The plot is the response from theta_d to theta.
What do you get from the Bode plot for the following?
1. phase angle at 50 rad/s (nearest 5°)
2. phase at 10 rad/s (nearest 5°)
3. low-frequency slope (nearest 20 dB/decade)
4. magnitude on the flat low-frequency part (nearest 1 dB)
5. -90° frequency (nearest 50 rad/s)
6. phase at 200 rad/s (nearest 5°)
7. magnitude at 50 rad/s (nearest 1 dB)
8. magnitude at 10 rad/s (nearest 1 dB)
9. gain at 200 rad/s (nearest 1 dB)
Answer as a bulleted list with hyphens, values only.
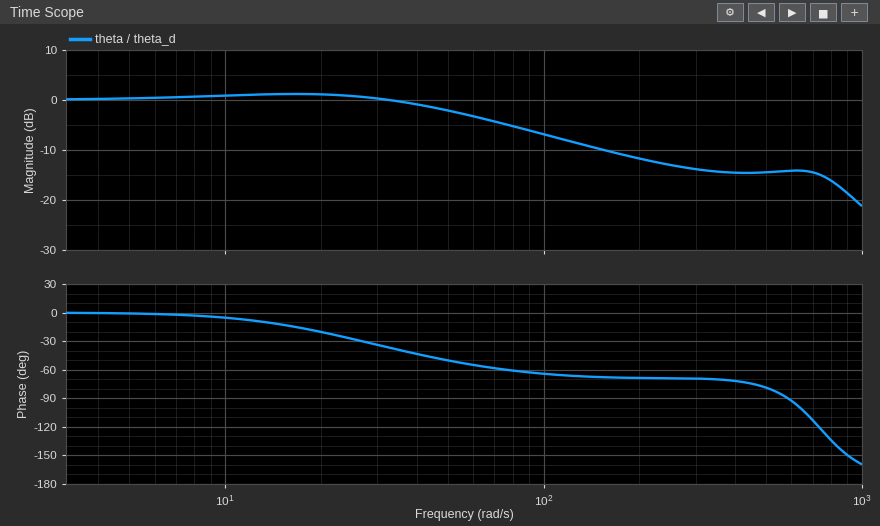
- -50°
- -5°
- 0 dB/decade
- 0 dB
- 600 rad/s
- -70°
- -2 dB
- 1 dB
- -12 dB
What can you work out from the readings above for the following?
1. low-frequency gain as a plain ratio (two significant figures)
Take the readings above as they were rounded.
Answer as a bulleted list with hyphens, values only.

- 1.0
